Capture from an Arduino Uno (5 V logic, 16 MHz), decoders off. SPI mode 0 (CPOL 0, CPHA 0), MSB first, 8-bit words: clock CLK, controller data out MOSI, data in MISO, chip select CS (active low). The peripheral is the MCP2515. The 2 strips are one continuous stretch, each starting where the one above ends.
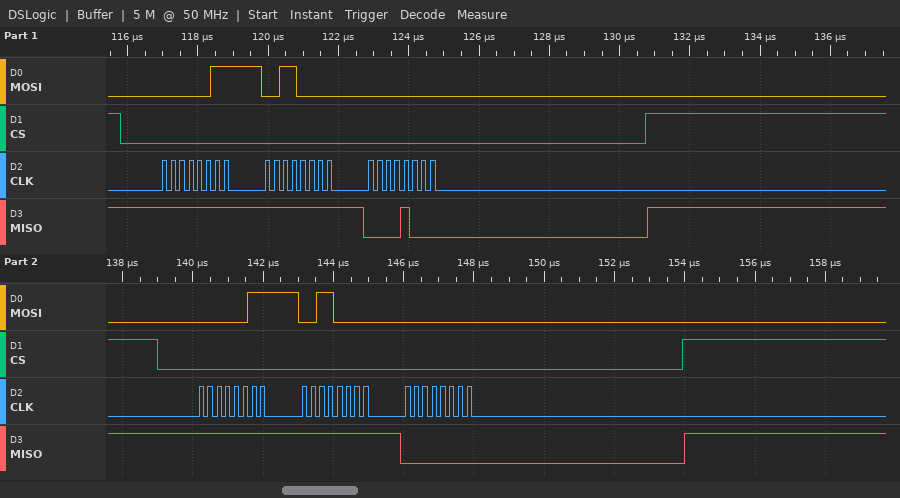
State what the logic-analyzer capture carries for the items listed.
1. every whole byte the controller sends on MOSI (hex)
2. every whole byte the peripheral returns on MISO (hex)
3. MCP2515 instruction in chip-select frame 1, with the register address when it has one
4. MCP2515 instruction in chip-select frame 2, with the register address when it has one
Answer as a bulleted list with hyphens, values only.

- 03 30 00 03 30 00
- FF FF 08 FF FF 00
- READ 0x30
- READ 0x30
